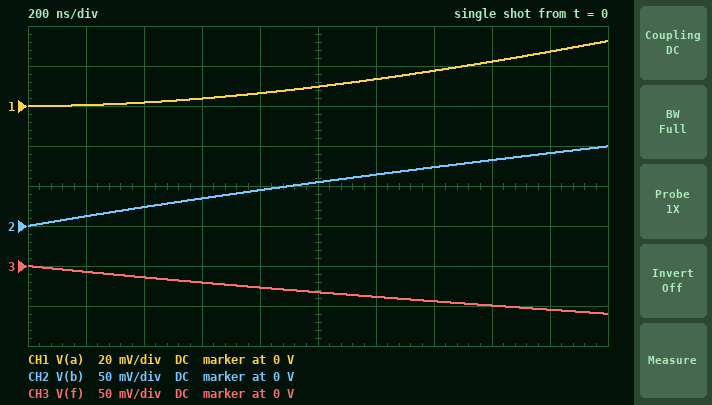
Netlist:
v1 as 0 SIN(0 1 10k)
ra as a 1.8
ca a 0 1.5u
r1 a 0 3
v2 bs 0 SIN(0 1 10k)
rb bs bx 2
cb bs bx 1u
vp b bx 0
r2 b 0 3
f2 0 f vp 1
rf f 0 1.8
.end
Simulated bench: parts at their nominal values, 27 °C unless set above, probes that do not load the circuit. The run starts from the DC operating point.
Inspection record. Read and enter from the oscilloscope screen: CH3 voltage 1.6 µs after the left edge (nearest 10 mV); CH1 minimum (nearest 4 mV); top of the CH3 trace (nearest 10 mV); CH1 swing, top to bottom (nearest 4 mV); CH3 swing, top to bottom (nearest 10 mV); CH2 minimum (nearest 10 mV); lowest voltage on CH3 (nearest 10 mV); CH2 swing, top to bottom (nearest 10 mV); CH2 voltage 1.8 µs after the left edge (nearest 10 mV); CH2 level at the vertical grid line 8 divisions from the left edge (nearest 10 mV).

-50 mV
0 V
0 V
32 mV
60 mV
0 V
-60 mV
100 mV
90 mV
80 mV
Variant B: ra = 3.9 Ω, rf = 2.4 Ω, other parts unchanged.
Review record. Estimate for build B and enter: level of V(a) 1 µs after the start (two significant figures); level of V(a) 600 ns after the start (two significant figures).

4.7 mV
1.8 mV
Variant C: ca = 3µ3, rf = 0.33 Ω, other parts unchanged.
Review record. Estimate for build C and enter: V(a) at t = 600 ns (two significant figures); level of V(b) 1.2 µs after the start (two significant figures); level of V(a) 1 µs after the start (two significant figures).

1.8 mV
64 mV
4.8 mV
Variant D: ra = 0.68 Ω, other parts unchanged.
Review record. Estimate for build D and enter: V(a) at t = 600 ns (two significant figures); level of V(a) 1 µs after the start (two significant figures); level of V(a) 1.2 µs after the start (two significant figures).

8.8 mV
21 mV
29 mV
